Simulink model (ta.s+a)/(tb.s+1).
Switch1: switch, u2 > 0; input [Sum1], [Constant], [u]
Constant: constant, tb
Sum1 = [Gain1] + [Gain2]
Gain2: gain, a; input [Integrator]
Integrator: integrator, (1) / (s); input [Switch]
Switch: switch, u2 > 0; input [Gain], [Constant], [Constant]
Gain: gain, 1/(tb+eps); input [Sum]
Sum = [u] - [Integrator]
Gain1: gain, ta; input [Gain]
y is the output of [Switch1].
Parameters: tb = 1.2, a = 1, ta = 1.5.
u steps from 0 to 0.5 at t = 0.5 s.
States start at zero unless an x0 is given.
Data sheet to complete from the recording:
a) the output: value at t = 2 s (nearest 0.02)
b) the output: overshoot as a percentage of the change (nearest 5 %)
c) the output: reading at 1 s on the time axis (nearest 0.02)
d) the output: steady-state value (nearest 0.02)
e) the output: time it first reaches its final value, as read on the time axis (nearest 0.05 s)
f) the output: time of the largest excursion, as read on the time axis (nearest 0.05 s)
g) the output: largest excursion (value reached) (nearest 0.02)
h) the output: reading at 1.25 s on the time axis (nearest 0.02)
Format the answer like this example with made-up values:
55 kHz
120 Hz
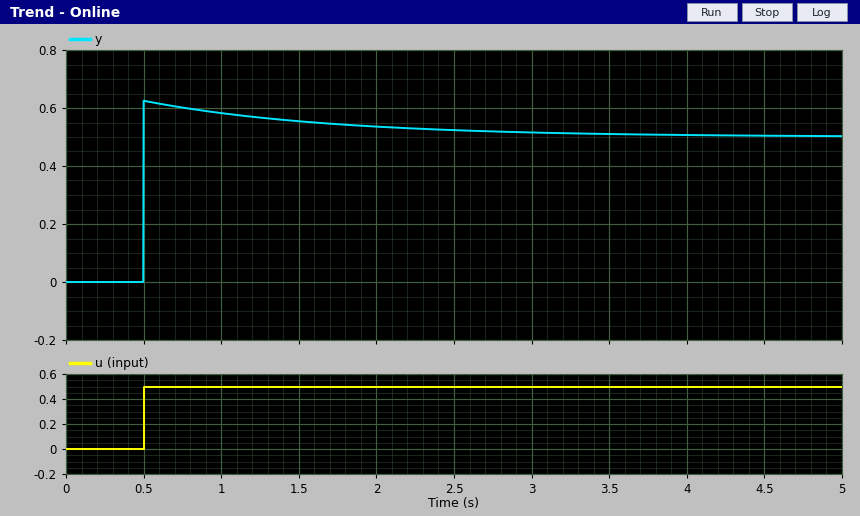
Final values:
0.54
25 %
0.58
0.50
0.50 s
0.50 s
0.62
0.56
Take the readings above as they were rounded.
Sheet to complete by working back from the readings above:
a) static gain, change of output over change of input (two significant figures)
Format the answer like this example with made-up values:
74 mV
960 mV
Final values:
1.0
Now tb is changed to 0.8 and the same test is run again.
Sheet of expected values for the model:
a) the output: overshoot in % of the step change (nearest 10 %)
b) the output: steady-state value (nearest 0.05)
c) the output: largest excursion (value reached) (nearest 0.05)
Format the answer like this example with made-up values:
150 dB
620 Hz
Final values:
90 %
0.50
0.95
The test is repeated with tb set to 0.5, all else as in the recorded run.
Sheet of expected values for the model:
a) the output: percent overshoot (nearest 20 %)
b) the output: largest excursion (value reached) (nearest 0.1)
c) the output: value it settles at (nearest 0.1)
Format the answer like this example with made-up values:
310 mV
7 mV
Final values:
200 %
1.5
0.5
